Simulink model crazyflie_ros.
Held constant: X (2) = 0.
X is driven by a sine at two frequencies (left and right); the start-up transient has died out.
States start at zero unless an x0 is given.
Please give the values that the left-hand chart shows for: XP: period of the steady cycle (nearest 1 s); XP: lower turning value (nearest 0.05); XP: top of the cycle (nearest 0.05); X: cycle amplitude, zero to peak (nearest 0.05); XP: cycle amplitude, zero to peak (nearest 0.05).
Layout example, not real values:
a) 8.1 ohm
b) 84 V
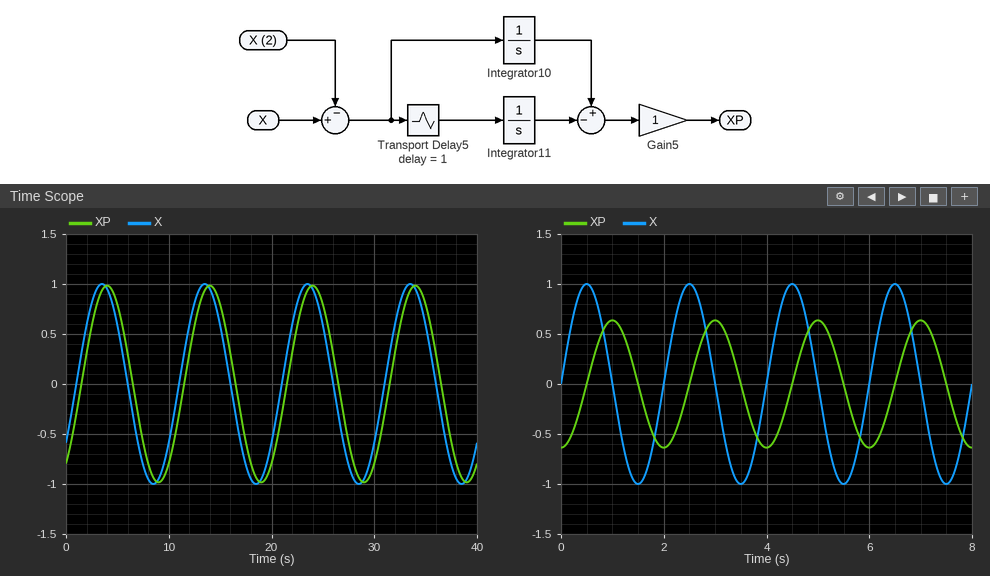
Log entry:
a) 10 s
b) -1.00
c) 1.00
d) 1.00
e) 1.00
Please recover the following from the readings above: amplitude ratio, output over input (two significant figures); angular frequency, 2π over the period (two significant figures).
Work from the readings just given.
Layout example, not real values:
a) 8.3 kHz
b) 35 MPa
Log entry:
a) 1.0
b) 0.63 rad/s
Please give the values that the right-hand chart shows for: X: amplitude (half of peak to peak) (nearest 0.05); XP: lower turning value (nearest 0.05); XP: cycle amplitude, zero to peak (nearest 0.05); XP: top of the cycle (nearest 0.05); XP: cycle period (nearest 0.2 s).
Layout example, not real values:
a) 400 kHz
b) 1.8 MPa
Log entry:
a) 1.00
b) -0.65
c) 0.65
d) 0.65
e) 2.0 s
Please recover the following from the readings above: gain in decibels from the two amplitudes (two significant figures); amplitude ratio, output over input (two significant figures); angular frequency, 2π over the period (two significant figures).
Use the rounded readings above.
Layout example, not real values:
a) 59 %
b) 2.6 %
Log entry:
a) -3.7 dB
b) 0.65
c) 3.1 rad/s
